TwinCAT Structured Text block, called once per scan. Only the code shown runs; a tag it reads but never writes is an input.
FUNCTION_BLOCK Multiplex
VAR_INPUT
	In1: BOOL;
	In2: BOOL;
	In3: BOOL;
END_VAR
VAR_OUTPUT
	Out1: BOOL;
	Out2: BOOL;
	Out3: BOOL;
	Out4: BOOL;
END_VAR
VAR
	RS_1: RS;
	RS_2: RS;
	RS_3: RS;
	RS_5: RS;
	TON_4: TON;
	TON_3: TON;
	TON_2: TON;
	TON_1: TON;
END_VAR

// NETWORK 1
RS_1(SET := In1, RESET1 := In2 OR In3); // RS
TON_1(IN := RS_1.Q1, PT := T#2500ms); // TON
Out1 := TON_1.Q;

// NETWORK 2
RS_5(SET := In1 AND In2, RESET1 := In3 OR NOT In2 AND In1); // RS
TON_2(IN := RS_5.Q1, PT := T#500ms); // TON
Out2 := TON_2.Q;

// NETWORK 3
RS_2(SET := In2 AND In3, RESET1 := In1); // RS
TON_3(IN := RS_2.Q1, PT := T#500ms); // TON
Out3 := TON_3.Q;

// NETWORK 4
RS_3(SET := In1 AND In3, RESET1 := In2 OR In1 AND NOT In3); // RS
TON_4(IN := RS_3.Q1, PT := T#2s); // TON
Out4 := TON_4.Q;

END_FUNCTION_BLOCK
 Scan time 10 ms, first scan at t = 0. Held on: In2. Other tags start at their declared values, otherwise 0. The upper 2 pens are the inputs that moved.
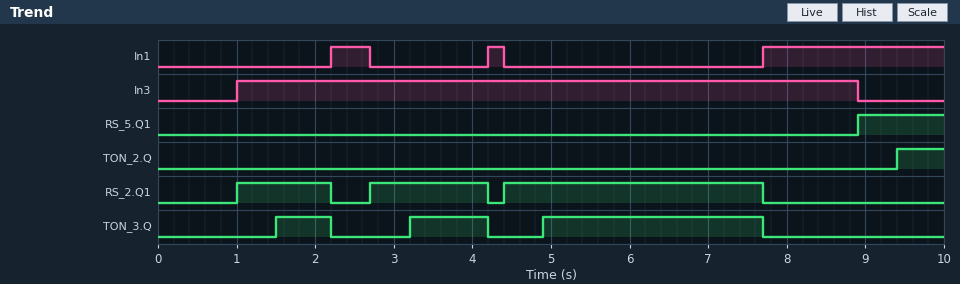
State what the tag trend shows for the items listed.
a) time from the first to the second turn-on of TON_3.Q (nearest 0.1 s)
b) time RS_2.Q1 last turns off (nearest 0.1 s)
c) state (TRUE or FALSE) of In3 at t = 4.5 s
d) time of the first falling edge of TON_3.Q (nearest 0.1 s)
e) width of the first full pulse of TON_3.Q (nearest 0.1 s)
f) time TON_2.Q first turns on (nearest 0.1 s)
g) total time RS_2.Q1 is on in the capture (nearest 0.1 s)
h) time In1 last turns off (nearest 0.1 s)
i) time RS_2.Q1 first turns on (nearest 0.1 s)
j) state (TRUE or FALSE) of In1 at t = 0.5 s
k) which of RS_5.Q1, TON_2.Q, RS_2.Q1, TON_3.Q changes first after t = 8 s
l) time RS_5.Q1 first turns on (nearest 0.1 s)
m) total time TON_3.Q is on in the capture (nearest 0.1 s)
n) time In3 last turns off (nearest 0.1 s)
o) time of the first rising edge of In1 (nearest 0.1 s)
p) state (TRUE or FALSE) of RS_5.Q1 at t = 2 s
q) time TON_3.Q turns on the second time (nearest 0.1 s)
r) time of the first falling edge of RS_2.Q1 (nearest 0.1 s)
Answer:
1.7 s
7.7 s
TRUE
2.2 s
0.7 s
9.4 s
6.0 s
4.4 s
1.0 s
FALSE
RS_5.Q1
8.9 s
4.5 s
8.9 s
2.2 s
FALSE
3.2 s
2.2 s
